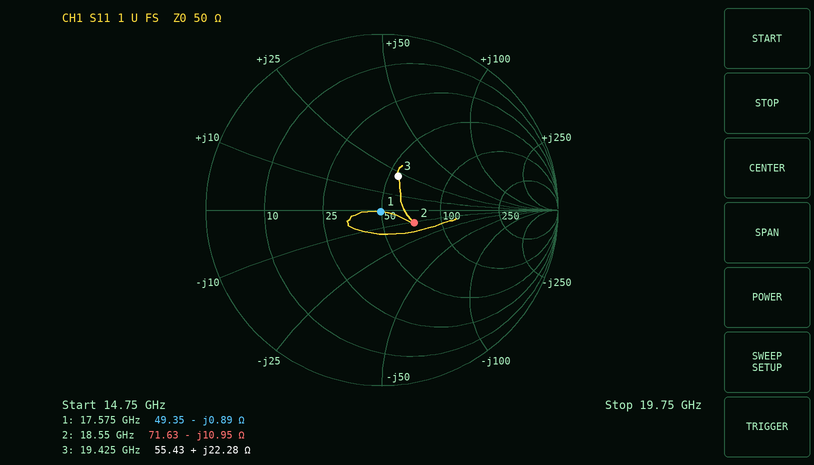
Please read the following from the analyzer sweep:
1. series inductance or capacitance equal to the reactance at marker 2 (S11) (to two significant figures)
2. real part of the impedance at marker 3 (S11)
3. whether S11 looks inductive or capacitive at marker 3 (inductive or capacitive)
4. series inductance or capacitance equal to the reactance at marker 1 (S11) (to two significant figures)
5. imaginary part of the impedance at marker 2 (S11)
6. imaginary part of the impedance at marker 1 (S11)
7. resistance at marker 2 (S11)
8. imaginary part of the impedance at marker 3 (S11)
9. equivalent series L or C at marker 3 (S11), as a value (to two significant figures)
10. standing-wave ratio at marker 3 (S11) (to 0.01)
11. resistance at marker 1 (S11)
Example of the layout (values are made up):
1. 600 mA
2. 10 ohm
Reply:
1. 780 fF
2. 55.43 Ω
3. inductive
4. 10 pF
5. -10.95 Ω
6. -0.89 Ω
7. 71.63 Ω
8. +22.28 Ω
9. 180 pH
10. 1.54
11. 49.35 Ω
